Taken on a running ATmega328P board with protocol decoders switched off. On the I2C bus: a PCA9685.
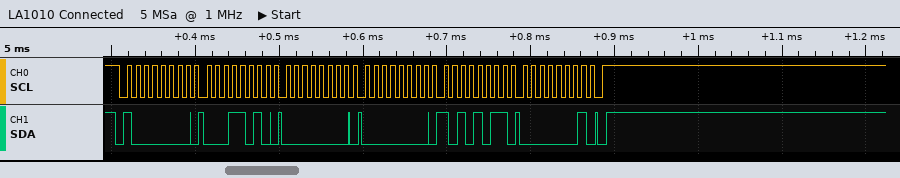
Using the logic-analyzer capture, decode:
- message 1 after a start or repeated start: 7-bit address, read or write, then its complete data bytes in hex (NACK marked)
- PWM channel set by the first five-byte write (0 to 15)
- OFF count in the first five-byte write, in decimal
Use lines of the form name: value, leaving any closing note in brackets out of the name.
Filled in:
message 1 after a start or repeated start: 7-bit address, read or write, then its complete data bytes in hex: 0x40 write: 1A 00 00 AB 01
PWM channel set by the first five-byte write: 5
OFF count in the first five-byte write, in decimal: 427
